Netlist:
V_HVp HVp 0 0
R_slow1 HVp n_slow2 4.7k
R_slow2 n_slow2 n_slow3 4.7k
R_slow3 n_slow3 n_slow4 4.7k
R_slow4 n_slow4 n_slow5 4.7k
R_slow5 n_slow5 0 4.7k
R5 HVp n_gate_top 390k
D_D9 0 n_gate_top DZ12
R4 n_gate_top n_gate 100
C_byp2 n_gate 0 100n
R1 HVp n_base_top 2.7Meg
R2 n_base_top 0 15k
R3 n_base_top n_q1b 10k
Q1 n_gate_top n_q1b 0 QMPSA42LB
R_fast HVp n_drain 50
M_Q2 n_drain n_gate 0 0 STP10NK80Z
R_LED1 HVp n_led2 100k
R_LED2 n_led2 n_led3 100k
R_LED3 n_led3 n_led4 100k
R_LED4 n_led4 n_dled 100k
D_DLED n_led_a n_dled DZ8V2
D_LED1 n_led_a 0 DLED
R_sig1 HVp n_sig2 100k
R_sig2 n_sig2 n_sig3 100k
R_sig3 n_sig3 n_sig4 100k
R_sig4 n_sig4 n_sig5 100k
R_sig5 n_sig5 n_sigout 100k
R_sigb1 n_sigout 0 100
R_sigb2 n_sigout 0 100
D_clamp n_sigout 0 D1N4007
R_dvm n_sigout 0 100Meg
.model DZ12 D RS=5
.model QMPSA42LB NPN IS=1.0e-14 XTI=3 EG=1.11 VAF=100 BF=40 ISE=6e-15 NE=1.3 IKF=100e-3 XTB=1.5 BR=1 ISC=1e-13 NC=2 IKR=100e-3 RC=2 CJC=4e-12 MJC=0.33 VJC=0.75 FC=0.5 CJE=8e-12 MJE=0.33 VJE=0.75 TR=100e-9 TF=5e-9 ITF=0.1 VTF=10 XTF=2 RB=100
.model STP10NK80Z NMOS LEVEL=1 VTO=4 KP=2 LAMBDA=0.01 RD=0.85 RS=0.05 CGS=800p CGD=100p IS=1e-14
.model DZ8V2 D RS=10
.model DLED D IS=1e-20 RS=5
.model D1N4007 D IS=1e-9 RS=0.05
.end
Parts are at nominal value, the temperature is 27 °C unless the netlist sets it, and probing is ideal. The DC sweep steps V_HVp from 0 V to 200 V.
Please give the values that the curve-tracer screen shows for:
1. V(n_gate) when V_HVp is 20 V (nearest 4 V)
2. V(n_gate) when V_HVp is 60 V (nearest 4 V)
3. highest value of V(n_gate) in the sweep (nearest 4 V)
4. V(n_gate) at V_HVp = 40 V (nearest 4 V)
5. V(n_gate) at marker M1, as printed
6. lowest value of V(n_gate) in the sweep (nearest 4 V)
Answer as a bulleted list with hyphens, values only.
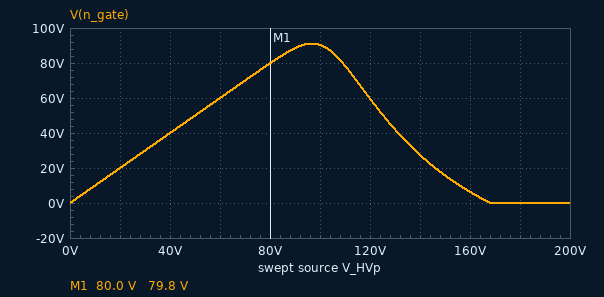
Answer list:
- 20 V
- 60 V
- 92 V
- 40 V
- 79.8 V
- 0 V
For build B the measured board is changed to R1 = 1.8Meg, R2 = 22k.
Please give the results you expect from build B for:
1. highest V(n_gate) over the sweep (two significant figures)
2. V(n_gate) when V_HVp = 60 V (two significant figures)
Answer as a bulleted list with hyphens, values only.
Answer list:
- 41 V
- 4.6 V
